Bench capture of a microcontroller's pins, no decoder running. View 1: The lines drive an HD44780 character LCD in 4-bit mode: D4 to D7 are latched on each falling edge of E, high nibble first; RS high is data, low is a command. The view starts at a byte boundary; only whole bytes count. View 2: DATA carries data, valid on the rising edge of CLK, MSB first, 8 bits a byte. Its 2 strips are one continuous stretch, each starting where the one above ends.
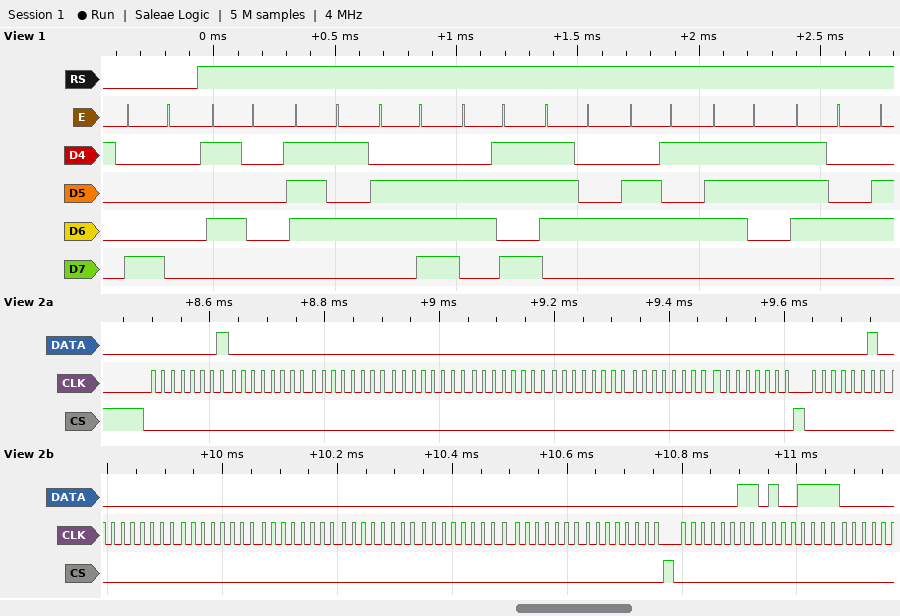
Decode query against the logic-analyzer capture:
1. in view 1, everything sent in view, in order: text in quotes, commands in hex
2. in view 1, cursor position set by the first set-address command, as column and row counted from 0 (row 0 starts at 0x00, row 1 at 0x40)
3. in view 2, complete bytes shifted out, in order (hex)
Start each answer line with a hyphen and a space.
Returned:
- 0x80 "Punktest"
- column 0, row 0
- 01 00 00 00 00 00 00 00 02 00 00 00 00 00 00 00 03 4F
